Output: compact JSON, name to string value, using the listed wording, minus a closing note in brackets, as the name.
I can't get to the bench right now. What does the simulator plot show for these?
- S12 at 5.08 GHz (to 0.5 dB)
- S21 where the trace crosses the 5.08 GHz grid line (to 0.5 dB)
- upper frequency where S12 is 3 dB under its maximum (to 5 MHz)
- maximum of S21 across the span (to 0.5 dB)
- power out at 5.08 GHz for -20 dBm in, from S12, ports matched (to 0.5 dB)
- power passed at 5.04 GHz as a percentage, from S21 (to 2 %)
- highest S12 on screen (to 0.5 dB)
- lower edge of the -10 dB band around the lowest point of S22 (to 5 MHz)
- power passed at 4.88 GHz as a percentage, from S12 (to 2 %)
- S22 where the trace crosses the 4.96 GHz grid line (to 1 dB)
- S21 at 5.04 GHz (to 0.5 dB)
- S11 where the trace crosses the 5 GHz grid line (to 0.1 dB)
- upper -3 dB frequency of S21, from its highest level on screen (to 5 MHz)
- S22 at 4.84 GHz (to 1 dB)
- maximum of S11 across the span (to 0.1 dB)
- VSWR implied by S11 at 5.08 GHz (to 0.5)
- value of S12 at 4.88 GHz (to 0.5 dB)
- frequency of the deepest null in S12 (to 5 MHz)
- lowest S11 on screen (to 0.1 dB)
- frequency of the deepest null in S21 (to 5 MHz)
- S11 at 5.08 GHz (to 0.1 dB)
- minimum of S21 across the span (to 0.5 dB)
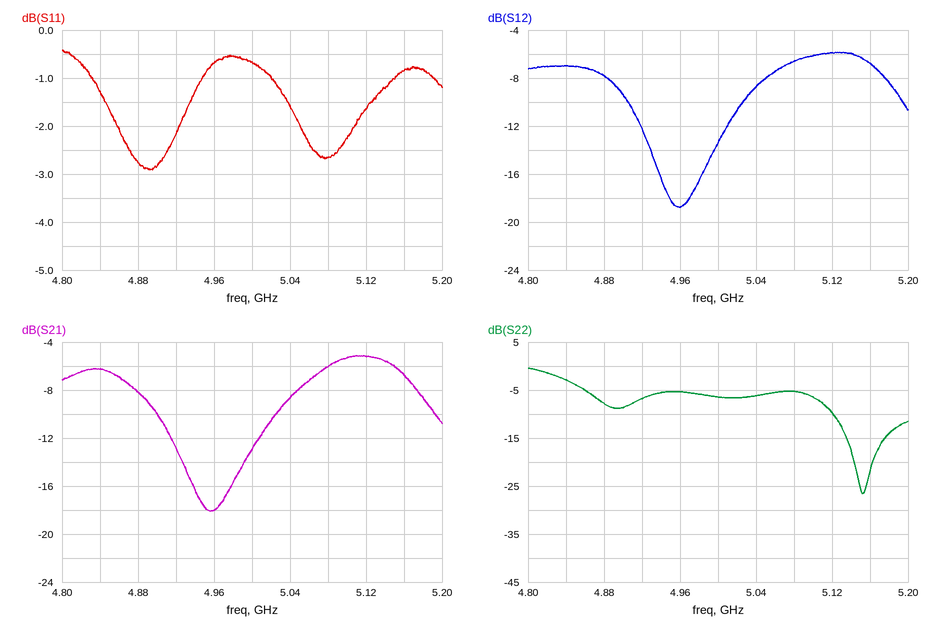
{"S12 at 5.08 GHz": "-6.5 dB", "S21 where the trace crosses the 5.08 GHz grid line": "-6.0 dB", "upper frequency where S12 is 3 dB under its maximum": "5.185 GHz", "maximum of S21 across the span": "-5.0 dB", "power out at 5.08 GHz for -20 dBm in, from S12, ports matched": "-26.5 dBm", "power passed at 5.04 GHz as a percentage, from S21": "14 %", "highest S12 on screen": "-6.0 dB", "lower edge of the -10 dB band around the lowest point of S22": "5.120 GHz", "power passed at 4.88 GHz as a percentage, from S12": "16 %", "S22 where the trace crosses the 4.96 GHz grid line": "-5 dB", "S21 at 5.04 GHz": "-8.5 dB", "S11 where the trace crosses the 5 GHz grid line": "-0.7 dB", "upper -3 dB frequency of S21, from its highest level on screen": "5.175 GHz", "S22 at 4.84 GHz": "-3 dB", "maximum of S11 across the span": "-0.4 dB", "VSWR implied by S11 at 5.08 GHz": "6.5", "value of S12 at 4.88 GHz": "-8.0 dB", "frequency of the deepest null in S12": "4.960 GHz", "lowest S11 on screen": "-2.9 dB", "frequency of the deepest null in S21": "4.955 GHz", "S11 at 5.08 GHz": "-2.7 dB", "minimum of S21 across the span": "-18.0 dB"}
